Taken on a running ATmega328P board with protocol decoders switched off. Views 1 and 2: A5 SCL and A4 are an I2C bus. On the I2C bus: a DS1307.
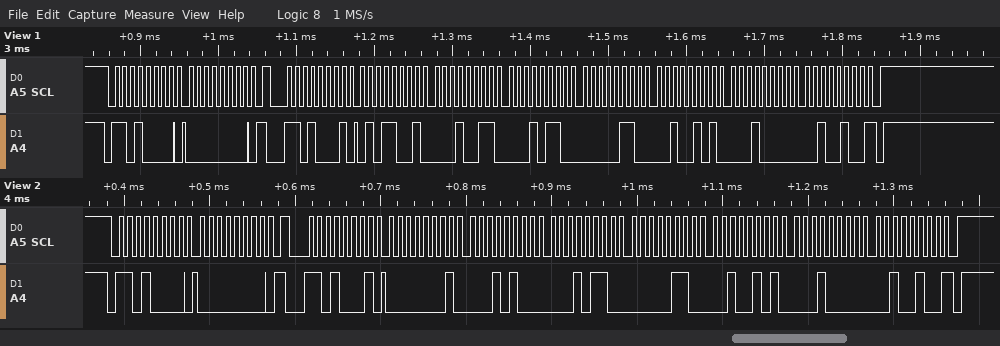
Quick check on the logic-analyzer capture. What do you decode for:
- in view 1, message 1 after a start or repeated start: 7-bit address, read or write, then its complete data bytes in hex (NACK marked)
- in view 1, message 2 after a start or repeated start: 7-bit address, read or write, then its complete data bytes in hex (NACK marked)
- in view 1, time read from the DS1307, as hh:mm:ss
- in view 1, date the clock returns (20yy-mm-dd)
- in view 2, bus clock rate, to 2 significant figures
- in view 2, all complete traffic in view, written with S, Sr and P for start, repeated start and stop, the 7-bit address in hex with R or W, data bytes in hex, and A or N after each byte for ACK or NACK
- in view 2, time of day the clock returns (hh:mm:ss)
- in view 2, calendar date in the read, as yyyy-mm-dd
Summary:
0x68 write: 00
0x68 read: 59 13 16 06 25 10 24 NACK
16:13:59
2024-10-25
100 kHz
S 68W A 00 A Sr 68R A 01 A 14 A 16 A 06 A 25 A 10 A 24 N P
16:14:01
2024-10-25
